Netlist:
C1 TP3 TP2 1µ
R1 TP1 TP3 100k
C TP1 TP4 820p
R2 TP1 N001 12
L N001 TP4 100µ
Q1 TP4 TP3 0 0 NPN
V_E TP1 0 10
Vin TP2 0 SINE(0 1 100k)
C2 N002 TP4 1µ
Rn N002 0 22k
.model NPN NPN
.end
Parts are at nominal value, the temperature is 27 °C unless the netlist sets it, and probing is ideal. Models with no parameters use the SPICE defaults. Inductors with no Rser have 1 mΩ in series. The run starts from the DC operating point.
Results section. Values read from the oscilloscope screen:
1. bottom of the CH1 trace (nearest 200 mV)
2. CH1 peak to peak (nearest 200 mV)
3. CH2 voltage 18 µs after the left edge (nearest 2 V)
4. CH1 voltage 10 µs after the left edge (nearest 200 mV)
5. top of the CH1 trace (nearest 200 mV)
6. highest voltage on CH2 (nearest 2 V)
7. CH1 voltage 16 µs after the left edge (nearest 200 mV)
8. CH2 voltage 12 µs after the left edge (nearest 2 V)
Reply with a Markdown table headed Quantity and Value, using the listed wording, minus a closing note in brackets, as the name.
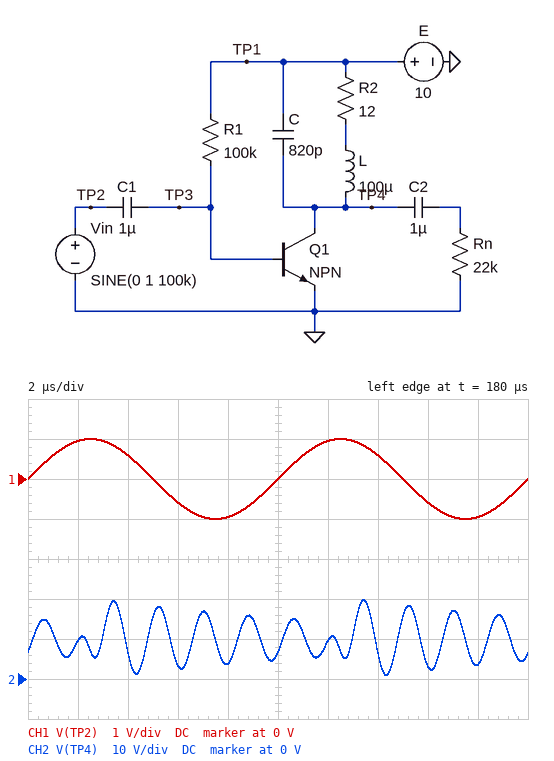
| Quantity | Value |
|---|---|
| bottom of the CH1 trace | -1.0 V |
| CH1 peak to peak | 2.0 V |
| CH2 voltage 18 µs after the left edge | 4 V |
| CH1 voltage 10 µs after the left edge | 0 V |
| top of the CH1 trace | 1.0 V |
| highest voltage on CH2 | 20 V |
| CH1 voltage 16 µs after the left edge | -600 mV |
| CH2 voltage 12 µs after the left edge | 10 V |
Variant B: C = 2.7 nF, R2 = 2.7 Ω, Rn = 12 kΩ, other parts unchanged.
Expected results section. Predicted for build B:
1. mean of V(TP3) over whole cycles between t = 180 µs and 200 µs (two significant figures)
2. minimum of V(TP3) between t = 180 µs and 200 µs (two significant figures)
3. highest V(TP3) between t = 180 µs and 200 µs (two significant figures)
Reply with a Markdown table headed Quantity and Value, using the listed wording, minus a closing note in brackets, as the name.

| Quantity | Value |
|---|---|
| mean of V(TP3) over whole cycles between t = 180 µs and 200 µs | -180 mV |
| minimum of V(TP3) between t = 180 µs and 200 µs | -1.2 V |
| highest V(TP3) between t = 180 µs and 200 µs | 820 mV |
